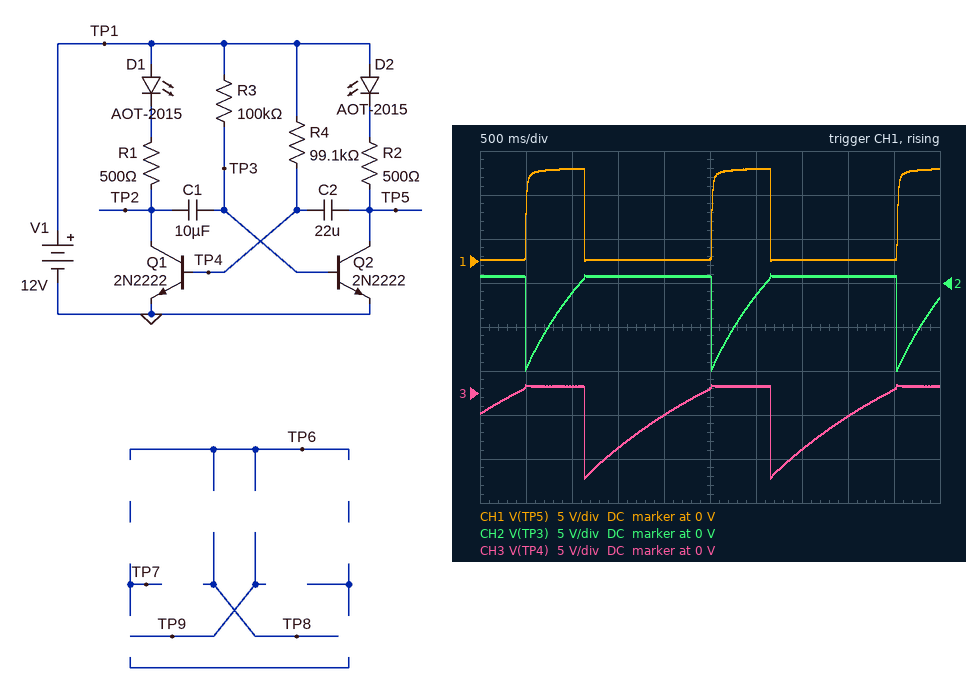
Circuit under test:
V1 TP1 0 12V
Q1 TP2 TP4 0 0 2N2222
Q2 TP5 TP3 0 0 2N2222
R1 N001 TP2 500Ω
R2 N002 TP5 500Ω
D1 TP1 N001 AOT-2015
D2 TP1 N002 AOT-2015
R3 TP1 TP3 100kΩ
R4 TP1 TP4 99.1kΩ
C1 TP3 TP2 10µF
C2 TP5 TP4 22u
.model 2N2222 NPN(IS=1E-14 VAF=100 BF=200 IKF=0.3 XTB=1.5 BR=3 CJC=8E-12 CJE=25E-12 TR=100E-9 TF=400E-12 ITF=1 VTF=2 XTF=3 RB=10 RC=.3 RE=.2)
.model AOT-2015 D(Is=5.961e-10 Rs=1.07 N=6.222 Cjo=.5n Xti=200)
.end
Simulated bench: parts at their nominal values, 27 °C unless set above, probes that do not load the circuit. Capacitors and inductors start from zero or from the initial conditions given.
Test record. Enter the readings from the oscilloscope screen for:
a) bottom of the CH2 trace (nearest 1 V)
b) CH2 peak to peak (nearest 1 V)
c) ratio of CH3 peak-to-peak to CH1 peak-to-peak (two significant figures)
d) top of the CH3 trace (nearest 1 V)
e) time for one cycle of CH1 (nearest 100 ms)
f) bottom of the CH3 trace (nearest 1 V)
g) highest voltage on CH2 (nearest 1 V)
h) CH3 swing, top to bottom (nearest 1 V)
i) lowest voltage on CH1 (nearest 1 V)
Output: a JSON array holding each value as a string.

["-10 V", "11 V", "1.0", "1 V", "2.0 s", "-10 V", "1 V", "11 V", "0 V"]
